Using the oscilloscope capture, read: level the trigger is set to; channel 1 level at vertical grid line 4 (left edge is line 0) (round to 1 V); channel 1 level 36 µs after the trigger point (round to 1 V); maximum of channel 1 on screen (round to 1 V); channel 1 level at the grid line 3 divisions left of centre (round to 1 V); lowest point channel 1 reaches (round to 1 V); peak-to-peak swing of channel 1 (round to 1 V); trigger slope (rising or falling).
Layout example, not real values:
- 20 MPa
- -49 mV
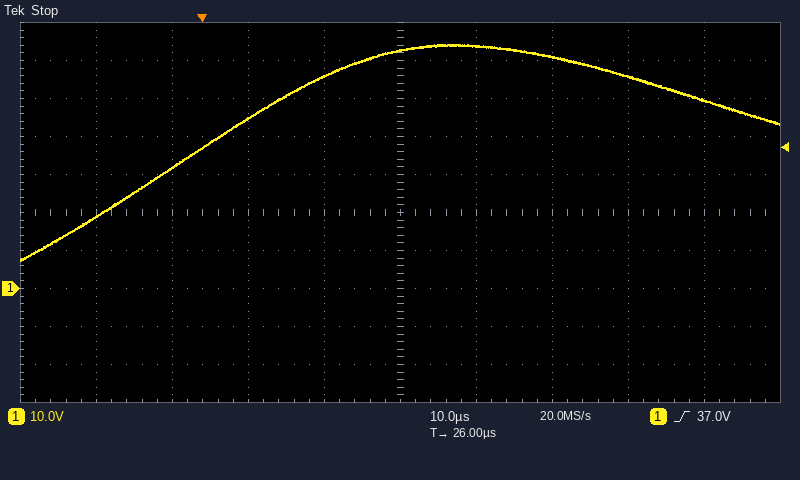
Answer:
- 37.0 V
- 56 V
- 64 V
- 64 V
- 32 V
- 7 V
- 57 V
- rising
